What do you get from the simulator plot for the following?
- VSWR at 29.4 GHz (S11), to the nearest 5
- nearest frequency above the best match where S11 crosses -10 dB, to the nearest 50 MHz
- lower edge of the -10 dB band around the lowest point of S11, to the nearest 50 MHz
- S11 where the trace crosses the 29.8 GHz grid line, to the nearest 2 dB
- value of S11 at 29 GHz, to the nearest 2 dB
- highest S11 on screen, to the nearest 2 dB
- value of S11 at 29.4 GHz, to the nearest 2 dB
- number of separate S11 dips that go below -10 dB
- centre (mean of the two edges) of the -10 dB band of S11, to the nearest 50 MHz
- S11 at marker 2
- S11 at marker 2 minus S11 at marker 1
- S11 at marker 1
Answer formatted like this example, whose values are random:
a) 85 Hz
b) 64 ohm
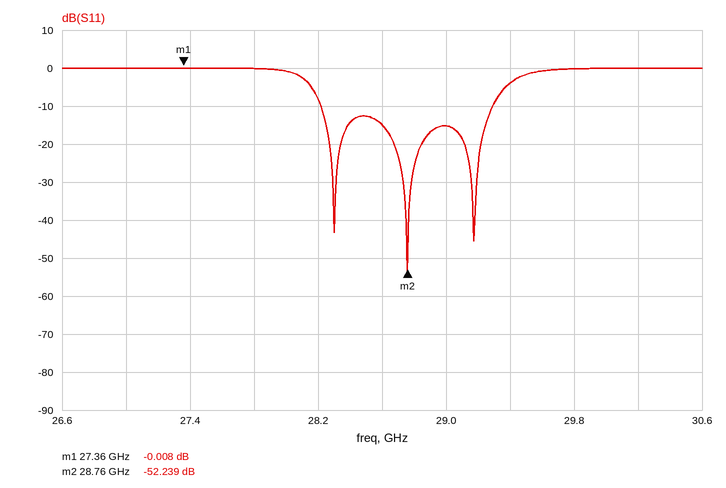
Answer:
a) 5
b) 29.30 GHz
c) 28.20 GHz
d) 0 dB
e) -16 dB
f) 0 dB
g) -4 dB
h) 3
i) 28.75 GHz
j) -52.239 dB
k) -52.231 dB
l) -0.008 dB
